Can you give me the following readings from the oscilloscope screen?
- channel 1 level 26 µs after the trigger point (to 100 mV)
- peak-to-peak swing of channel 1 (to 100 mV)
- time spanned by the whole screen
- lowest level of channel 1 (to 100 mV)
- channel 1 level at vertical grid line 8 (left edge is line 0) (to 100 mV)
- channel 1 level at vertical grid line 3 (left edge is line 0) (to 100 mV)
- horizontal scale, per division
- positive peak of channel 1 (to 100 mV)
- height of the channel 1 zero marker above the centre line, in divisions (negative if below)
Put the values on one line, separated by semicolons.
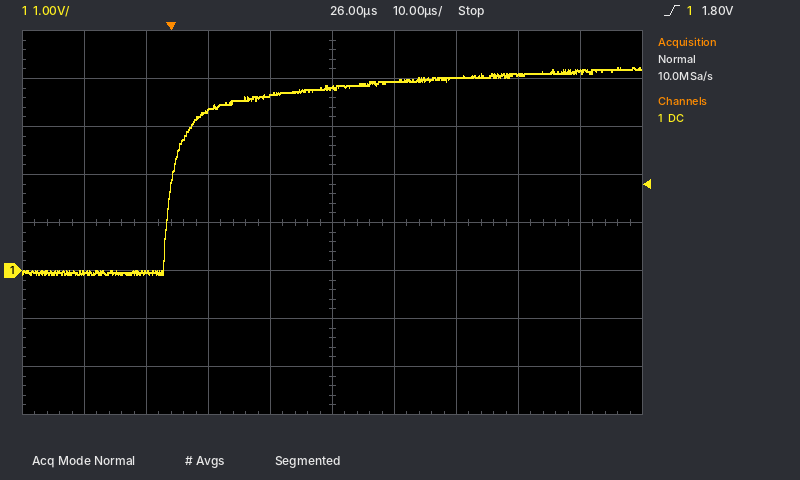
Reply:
3.8 V; 4.3 V; 100 µs; -100 mV; 4.1 V; 3.3 V; 10 µs; 4.2 V; -1.0 div
